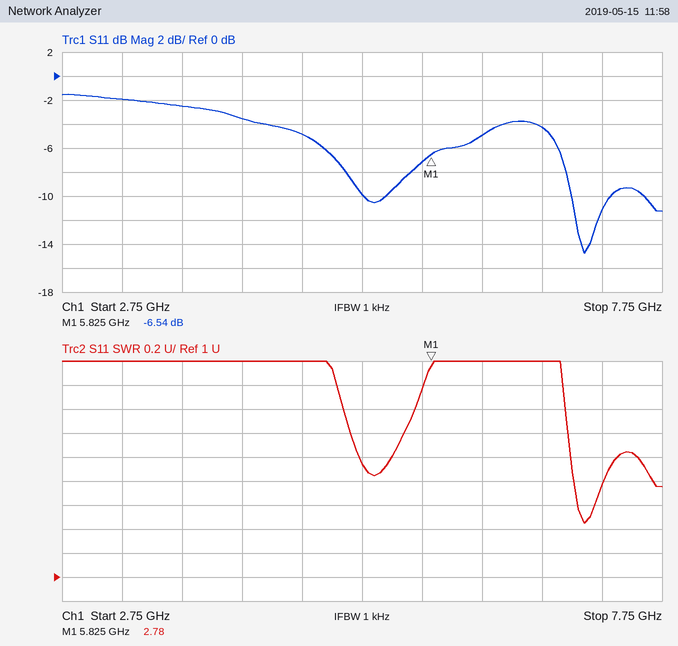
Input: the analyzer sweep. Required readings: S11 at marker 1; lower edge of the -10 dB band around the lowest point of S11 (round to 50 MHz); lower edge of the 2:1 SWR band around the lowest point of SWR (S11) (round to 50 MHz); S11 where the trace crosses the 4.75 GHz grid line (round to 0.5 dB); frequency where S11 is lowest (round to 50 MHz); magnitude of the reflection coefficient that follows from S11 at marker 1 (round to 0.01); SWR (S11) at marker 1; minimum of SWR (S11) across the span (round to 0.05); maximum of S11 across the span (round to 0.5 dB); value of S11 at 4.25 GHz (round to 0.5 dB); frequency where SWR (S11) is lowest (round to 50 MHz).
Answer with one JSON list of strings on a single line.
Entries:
["-6.54 dB", "7.00 GHz", "7.00 GHz", "-5.0 dB", "7.10 GHz", "0.47", "2.78", "1.45", "-1.5 dB", "-3.5 dB", "7.10 GHz"]
